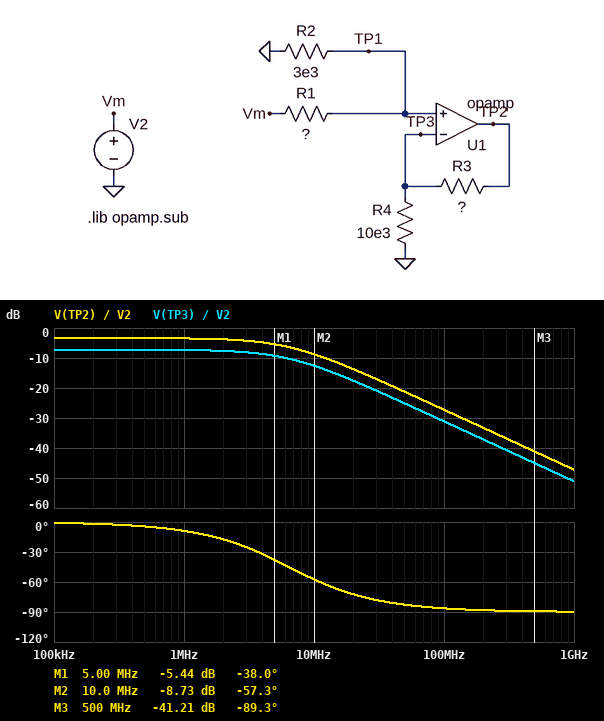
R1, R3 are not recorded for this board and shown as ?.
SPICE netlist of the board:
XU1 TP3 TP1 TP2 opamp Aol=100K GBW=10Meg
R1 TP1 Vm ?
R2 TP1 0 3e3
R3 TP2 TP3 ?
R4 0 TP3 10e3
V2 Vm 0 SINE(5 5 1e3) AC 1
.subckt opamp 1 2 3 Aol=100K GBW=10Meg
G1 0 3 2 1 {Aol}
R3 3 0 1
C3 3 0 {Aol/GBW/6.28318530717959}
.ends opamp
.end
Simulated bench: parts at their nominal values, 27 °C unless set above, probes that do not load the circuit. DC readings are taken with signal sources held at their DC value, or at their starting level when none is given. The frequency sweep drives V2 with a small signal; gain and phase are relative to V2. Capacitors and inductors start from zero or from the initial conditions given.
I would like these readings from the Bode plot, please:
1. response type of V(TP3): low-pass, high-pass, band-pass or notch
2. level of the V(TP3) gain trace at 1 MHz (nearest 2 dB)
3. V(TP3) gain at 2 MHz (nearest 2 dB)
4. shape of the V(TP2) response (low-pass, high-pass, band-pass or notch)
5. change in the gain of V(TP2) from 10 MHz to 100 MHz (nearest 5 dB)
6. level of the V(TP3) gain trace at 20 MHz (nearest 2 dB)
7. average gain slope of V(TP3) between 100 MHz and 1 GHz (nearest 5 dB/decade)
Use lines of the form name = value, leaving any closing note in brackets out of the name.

response type of V(TP3): low-pass, high-pass, band-pass or notch = low-pass
level of the V(TP3) gain trace at 1 MHz = -8 dB
V(TP3) gain at 2 MHz = -8 dB
shape of the V(TP2) response = low-pass
change in the gain of V(TP2) from 10 MHz to 100 MHz = -20 dB
level of the V(TP3) gain trace at 20 MHz = -18 dB
average gain slope of V(TP3) between 100 MHz and 1 GHz = -20 dB/decade
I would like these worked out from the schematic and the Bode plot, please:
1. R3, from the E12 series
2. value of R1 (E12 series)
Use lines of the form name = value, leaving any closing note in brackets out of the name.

R3, from the E12 series = 5.6 kΩ
value of R1 = 3.9 kΩ
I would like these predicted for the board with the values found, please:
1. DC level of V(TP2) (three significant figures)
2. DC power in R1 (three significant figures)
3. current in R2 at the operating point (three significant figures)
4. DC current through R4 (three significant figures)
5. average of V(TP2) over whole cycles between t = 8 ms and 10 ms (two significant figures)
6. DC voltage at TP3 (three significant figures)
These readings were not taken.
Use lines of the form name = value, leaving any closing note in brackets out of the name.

DC level of V(TP2) = 3.39 V
DC power in R1 = 2.05 mW
current in R2 at the operating point = 725 µA
DC current through R4 = 217 µA
average of V(TP2) over whole cycles between t = 8 ms and 10 ms = 3.4 V
DC voltage at TP3 = 2.17 V
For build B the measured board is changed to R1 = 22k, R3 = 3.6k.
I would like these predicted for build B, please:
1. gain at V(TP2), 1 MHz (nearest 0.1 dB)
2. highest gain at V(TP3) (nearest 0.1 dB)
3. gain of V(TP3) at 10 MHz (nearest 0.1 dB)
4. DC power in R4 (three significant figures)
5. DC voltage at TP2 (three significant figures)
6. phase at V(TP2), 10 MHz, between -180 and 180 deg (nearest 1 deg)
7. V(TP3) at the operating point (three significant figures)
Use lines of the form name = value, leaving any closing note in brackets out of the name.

gain at V(TP2), 1 MHz = -15.8 dB
highest gain at V(TP3) = -18.4 dB
gain of V(TP3) at 10 MHz = -23.0 dB
DC power in R4 = 36.0 µW
DC voltage at TP2 = 816 mV
phase at V(TP2), 10 MHz, between -180 and 180 deg = -54 deg
V(TP3) at the operating point = 600 mV
